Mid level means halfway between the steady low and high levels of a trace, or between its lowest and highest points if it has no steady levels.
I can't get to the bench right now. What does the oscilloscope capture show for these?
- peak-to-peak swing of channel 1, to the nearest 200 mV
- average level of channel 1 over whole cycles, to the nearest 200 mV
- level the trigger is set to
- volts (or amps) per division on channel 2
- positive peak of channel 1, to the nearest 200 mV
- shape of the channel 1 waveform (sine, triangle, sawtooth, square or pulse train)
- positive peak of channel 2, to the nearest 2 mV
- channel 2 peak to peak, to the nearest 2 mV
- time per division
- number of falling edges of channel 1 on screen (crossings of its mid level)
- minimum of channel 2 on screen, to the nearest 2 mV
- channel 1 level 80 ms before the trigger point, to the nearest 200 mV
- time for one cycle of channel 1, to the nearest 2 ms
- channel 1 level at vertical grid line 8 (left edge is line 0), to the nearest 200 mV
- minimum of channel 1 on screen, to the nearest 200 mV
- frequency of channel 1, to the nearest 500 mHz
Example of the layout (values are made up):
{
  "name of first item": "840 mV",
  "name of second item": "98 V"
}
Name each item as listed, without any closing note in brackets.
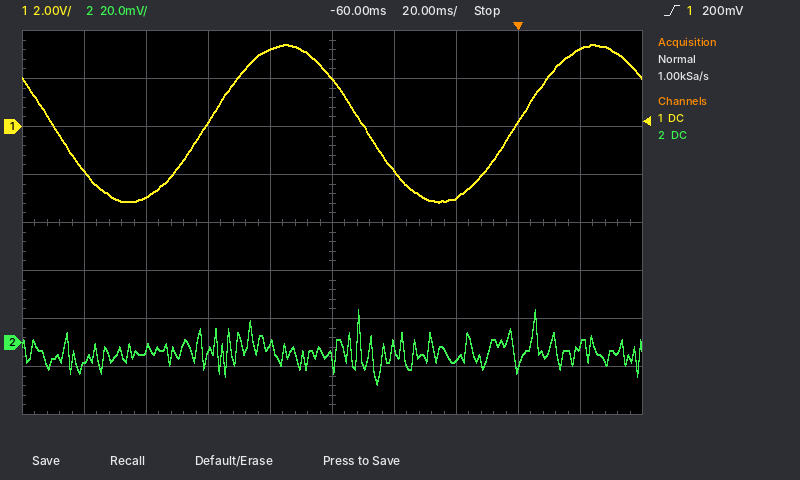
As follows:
{
  "peak-to-peak swing of channel 1, to the nearest 200 mV": "6.6 V",
  "average level of channel 1 over whole cycles, to the nearest 200 mV": "200 mV",
  "level the trigger is set to": "200 mV",
  "volts (or amps) per division on channel 2": "20 mV",
  "positive peak of channel 1, to the nearest 200 mV": "3.4 V",
  "shape of the channel 1 waveform": "sine",
  "positive peak of channel 2, to the nearest 2 mV": "14 mV",
  "channel 2 peak to peak, to the nearest 2 mV": "32 mV",
  "time per division": "20 ms",
  "number of falling edges of channel 1 on screen": "2",
  "minimum of channel 2 on screen, to the nearest 2 mV": "-18 mV",
  "channel 1 level 80 ms before the trigger point, to the nearest 200 mV": "3.2 V",
  "time for one cycle of channel 1, to the nearest 2 ms": "100 ms",
  "channel 1 level at vertical grid line 8 (left edge is line 0), to the nearest 200 mV": "200 mV",
  "minimum of channel 1 on screen, to the nearest 200 mV": "-3.2 V",
  "frequency of channel 1, to the nearest 500 mHz": "10.0 Hz"
}
